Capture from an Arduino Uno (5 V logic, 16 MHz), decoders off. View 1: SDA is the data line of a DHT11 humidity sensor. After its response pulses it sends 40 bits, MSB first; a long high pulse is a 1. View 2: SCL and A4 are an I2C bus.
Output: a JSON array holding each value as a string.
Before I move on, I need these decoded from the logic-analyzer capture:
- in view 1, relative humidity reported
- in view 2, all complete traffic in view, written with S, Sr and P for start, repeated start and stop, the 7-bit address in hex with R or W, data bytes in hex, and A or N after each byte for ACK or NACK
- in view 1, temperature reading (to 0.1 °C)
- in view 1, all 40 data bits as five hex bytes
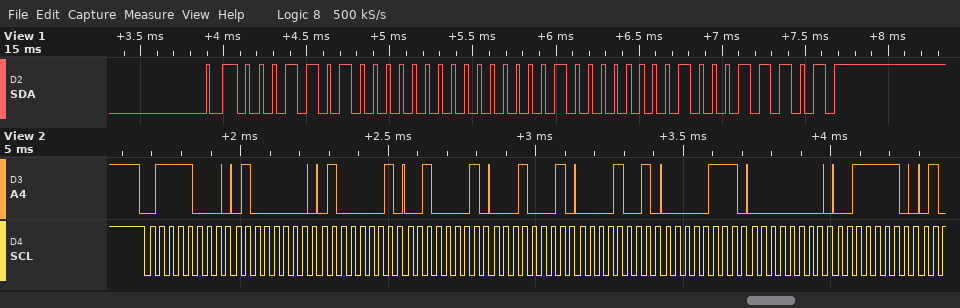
["26 %", "S 3CW A 40 A 41 A 21 A 11 A 09 A 07 A 00 A 3E A", "2.1 °C", "1A 00 02 01 1D"]
